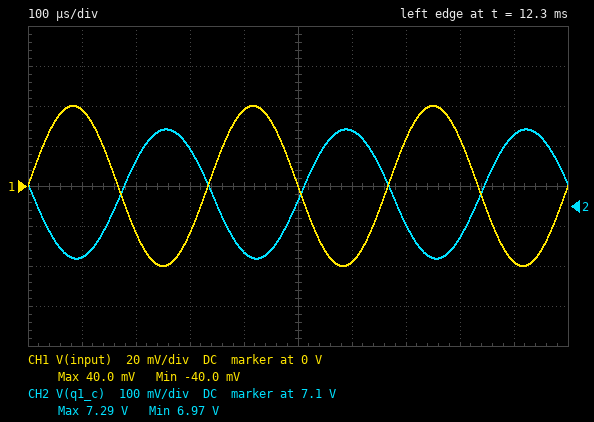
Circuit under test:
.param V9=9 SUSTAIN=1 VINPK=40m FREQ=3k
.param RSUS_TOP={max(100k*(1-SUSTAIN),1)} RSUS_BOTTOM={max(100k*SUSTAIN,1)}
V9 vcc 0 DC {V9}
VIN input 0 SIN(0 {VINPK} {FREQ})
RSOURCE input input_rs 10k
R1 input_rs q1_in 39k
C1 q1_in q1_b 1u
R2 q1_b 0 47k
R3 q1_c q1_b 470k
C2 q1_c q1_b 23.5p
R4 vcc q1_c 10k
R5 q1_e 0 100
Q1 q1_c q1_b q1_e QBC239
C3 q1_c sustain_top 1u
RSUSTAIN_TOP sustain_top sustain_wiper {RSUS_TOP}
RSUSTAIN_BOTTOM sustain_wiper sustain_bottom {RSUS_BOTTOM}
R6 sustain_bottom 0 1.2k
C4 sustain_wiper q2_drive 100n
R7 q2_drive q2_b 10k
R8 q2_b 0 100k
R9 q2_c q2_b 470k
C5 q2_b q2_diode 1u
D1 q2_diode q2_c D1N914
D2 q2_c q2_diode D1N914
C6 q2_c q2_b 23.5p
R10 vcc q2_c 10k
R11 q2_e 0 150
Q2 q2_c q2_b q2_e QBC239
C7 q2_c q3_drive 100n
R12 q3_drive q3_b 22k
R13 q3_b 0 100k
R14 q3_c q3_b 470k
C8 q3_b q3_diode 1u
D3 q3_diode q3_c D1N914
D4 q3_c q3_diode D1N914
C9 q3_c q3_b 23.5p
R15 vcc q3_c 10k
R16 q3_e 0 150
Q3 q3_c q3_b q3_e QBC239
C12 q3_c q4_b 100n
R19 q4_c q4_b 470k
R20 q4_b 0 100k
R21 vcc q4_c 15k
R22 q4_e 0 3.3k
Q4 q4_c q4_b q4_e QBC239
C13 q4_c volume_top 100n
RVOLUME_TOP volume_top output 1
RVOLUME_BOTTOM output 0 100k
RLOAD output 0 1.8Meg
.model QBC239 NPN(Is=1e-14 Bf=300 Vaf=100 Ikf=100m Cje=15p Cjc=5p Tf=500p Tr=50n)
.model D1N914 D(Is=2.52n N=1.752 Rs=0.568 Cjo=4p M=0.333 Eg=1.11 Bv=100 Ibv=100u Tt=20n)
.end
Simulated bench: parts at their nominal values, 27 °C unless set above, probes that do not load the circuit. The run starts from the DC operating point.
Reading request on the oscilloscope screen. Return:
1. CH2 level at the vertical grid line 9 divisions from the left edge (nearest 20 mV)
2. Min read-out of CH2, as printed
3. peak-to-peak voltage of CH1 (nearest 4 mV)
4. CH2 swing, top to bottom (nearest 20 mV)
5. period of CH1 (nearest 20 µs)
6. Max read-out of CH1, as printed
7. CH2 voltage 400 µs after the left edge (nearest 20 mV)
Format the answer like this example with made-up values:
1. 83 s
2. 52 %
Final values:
1. 7.28 V
2. 6.97 V
3. 80 mV
4. 320 mV
5. 340 µs
6. 40.0 mV
7. 6.98 V
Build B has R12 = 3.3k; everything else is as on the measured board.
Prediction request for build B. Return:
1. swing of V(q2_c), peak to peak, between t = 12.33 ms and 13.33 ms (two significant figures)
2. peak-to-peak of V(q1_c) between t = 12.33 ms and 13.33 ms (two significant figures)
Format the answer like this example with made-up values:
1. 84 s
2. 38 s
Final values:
1. 710 mV
2. 330 mV
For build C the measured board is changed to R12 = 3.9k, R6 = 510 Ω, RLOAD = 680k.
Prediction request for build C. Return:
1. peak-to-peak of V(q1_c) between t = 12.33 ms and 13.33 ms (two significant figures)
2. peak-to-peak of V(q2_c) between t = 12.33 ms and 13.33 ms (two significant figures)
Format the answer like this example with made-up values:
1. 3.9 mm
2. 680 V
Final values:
1. 330 mV
2. 710 mV
